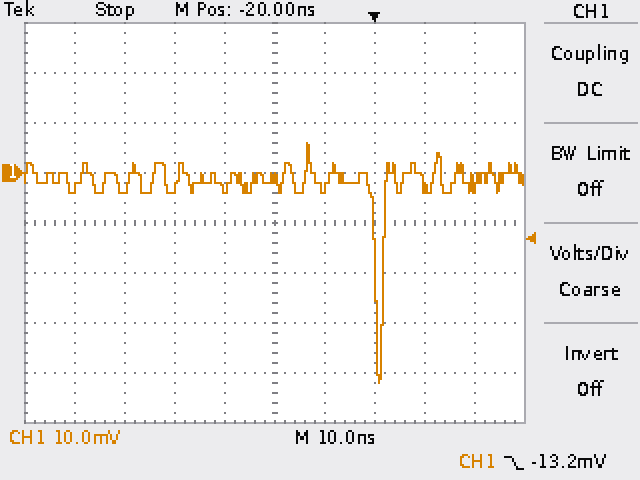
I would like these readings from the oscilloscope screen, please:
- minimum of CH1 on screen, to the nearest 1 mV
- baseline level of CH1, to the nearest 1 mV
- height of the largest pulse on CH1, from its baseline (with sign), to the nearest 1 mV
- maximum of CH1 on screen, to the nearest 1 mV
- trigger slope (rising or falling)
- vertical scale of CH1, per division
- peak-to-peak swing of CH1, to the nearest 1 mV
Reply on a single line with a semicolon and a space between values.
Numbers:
-42 mV; -1 mV; -41 mV; 6 mV; falling; 10 mV; 48 mV
